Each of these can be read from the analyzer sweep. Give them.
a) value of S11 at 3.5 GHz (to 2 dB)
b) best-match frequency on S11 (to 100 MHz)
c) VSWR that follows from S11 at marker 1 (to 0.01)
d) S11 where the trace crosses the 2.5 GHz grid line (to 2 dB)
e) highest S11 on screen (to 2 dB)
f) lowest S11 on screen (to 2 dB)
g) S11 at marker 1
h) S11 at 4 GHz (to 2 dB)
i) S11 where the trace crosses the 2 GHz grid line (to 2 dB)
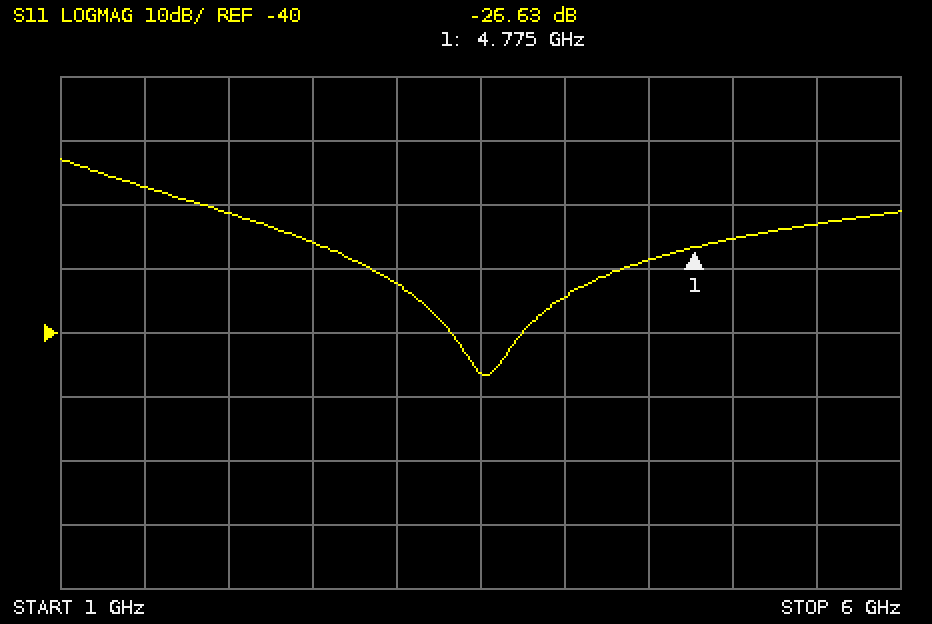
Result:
-46 dB
3.5 GHz
1.10
-26 dB
-12 dB
-46 dB
-26.63 dB
-34 dB
-22 dB
